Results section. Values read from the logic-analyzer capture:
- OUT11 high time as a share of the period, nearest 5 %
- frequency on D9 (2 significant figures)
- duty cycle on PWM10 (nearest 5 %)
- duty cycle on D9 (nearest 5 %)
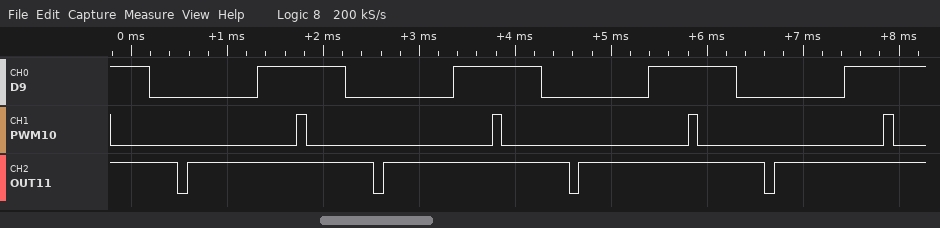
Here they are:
95 %
490 Hz
5 %
45 %
